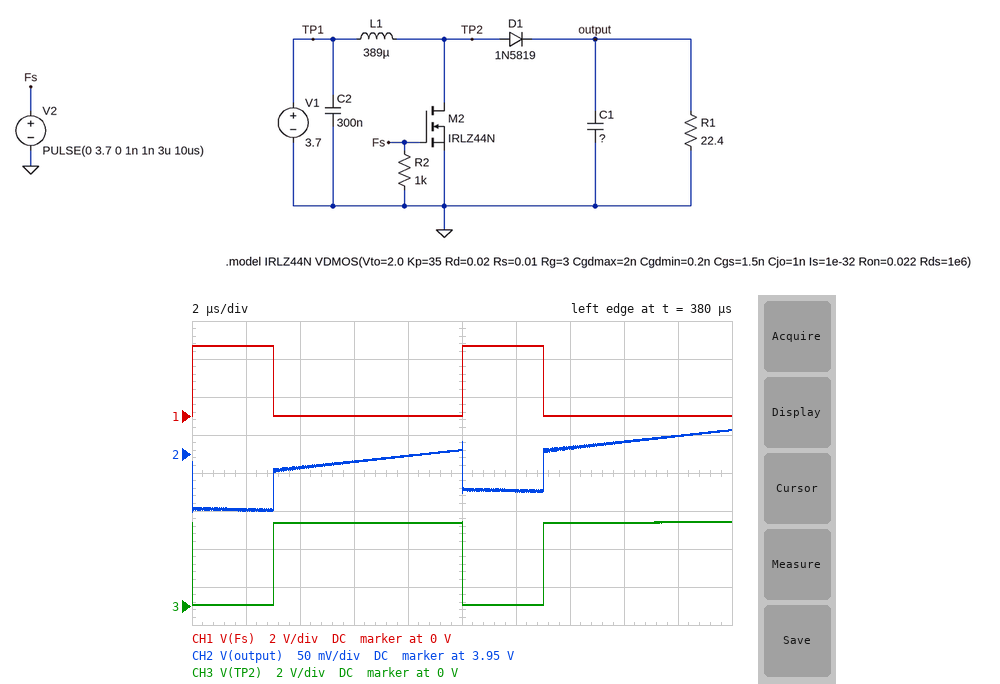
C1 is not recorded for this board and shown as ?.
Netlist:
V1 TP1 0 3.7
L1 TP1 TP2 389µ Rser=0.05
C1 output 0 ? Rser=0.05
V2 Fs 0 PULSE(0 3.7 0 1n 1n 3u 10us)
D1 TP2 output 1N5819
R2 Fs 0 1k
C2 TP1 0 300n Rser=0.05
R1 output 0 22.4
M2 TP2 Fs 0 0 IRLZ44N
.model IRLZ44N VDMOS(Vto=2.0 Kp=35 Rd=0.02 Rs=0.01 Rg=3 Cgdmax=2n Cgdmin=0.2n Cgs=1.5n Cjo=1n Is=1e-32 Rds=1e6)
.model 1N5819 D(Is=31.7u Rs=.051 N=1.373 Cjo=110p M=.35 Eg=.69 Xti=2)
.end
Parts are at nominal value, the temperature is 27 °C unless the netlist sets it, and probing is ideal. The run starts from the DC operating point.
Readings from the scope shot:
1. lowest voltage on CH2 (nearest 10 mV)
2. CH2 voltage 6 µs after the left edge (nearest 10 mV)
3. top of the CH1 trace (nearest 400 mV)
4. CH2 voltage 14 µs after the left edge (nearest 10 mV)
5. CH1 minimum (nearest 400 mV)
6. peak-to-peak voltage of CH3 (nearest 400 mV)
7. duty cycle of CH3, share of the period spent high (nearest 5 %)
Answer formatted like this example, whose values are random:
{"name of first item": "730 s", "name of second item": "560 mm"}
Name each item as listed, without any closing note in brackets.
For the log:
{"lowest voltage on CH2": "3.87 V", "CH2 voltage 6 µs after the left edge": "3.94 V", "top of the CH1 trace": "3.6 V", "CH2 voltage 14 µs after the left edge": "3.96 V", "CH1 minimum": "0 V", "peak-to-peak voltage of CH3": "4.4 V", "duty cycle of CH3, share of the period spent high": "70 %"}
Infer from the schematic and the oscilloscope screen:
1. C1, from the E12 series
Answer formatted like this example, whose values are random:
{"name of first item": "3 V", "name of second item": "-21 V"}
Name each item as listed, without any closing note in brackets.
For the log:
{"C1, from the E12 series": "220 µF"}
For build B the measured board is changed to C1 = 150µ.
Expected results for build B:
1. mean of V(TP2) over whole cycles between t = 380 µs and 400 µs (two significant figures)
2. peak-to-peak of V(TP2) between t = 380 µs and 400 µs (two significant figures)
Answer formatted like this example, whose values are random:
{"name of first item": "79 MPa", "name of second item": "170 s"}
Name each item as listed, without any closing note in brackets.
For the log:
{"mean of V(TP2) over whole cycles between t = 380 µs and 400 µs": "3.2 V", "peak-to-peak of V(TP2) between t = 380 µs and 400 µs": "4.6 V"}
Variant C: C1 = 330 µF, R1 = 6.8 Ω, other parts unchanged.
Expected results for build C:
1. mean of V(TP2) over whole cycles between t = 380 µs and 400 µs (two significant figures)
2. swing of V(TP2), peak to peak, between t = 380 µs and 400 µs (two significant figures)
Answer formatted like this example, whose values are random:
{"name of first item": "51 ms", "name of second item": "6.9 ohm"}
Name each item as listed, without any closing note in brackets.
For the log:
{"mean of V(TP2) over whole cycles between t = 380 µs and 400 µs": "2.9 V", "swing of V(TP2), peak to peak, between t = 380 µs and 400 µs": "4.1 V"}
